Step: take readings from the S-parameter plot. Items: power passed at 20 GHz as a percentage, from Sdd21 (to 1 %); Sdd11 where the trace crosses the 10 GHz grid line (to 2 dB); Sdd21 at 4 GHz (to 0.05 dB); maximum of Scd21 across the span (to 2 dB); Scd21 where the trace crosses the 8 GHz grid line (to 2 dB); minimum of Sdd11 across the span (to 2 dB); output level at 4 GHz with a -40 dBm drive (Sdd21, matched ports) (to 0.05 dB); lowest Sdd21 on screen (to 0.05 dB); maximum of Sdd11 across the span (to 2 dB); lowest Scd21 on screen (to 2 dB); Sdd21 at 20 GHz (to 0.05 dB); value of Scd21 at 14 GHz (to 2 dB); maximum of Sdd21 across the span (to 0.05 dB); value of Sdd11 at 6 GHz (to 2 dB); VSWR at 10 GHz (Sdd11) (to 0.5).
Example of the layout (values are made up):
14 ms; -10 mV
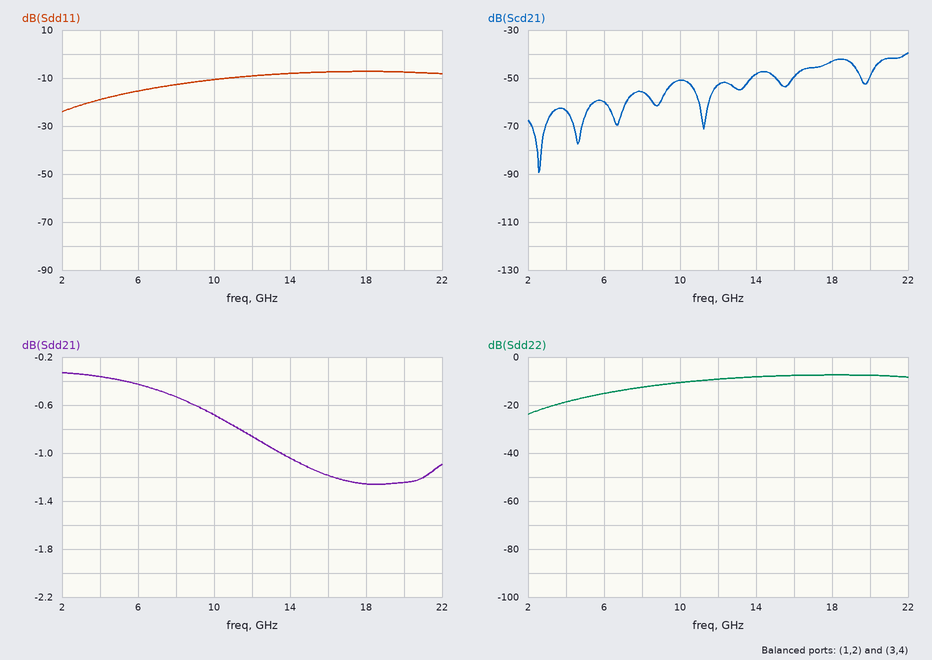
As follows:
75 %; -10 dB; -0.35 dB; -40 dB; -56 dB; -24 dB; -40.35 dBm; -1.25 dB; -8 dB; -90 dB; -1.25 dB; -48 dB; -0.35 dB; -16 dB; 2.0
